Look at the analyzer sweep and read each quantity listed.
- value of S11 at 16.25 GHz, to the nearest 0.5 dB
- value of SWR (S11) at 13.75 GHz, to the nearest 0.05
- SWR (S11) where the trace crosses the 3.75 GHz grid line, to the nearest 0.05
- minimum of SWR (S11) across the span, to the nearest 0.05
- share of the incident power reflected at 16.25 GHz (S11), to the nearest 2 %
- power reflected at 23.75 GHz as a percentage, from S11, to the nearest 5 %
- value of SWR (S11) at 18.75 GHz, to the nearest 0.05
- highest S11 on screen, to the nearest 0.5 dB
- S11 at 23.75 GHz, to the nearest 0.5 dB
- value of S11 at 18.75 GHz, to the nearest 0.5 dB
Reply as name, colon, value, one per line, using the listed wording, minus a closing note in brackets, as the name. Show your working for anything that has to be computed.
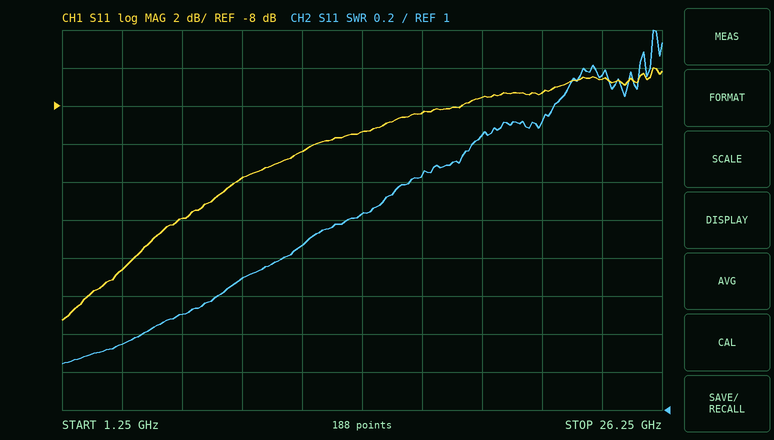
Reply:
value of S11 at 16.25 GHz, to the nearest 0.5 dB: -8.5 dB
value of SWR (S11) at 13.75 GHz, to the nearest 0.05: 2.05
SWR (S11) where the trace crosses the 3.75 GHz grid line, to the nearest 0.05: 1.35
minimum of SWR (S11) across the span, to the nearest 0.05: 1.25
share of the incident power reflected at 16.25 GHz (S11), to the nearest 2 %: 10^(-8.5/10) ≈ 14 %
power reflected at 23.75 GHz as a percentage, from S11, to the nearest 5 %: 10^(-6.5/10) ≈ 22.4 %, so 20 % to the nearest 5 %
value of SWR (S11) at 18.75 GHz, to the nearest 0.05: 2.45
highest S11 on screen, to the nearest 0.5 dB: -6.0 dB
S11 at 23.75 GHz, to the nearest 0.5 dB: -6.5 dB
value of S11 at 18.75 GHz, to the nearest 0.5 dB: -7.5 dB
